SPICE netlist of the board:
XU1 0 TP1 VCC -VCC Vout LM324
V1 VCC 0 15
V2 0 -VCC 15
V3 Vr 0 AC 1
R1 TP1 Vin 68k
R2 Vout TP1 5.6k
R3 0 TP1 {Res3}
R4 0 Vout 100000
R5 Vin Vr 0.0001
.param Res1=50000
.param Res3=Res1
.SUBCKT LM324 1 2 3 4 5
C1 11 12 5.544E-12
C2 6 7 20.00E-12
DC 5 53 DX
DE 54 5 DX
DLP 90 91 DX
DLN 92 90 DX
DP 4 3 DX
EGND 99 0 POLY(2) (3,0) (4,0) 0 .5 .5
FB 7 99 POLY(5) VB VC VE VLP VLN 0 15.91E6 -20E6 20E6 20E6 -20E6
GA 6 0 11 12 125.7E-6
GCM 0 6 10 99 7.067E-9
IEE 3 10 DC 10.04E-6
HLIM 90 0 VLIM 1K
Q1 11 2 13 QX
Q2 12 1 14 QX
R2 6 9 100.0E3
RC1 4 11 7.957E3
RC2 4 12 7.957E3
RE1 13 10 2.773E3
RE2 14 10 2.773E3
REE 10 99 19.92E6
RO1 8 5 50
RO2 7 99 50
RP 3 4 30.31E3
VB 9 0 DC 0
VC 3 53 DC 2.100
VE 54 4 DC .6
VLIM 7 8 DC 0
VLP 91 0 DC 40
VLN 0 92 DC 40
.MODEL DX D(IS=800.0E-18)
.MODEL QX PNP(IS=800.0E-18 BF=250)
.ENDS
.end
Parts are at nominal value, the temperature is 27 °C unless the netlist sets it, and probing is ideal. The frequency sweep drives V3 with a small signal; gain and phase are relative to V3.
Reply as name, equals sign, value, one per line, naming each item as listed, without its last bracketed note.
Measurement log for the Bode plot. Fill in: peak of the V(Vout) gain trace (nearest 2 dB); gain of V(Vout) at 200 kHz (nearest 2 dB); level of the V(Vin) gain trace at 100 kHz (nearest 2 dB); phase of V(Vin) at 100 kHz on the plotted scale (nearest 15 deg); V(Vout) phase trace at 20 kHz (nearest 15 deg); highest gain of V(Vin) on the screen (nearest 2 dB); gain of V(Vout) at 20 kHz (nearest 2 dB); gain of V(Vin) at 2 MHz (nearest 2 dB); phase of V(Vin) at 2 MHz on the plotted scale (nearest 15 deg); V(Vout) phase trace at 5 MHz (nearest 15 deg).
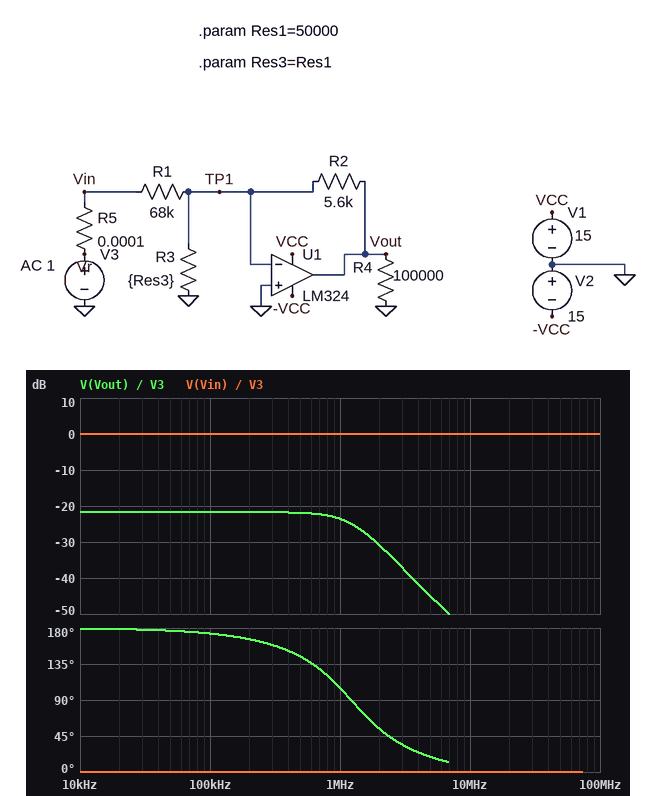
peak of the V(Vout) gain trace = -22 dB
gain of V(Vout) at 200 kHz = -22 dB
level of the V(Vin) gain trace at 100 kHz = 0 dB
phase of V(Vin) at 100 kHz on the plotted scale = 0 deg
V(Vout) phase trace at 20 kHz = 180 deg
highest gain of V(Vin) on the screen = 0 dB
gain of V(Vout) at 20 kHz = -22 dB
gain of V(Vin) at 2 MHz = 0 dB
phase of V(Vin) at 2 MHz on the plotted scale = 0 deg
V(Vout) phase trace at 5 MHz = 15 deg
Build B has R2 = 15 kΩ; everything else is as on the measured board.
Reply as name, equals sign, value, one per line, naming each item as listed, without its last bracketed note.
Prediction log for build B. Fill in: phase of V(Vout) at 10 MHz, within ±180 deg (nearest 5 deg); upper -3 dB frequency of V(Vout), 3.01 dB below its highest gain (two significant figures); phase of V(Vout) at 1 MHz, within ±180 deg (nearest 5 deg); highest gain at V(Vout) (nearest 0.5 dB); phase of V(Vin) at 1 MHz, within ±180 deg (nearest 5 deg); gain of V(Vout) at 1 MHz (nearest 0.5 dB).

phase of V(Vout) at 10 MHz, within ±180 deg = 10 deg
upper -3 dB frequency of V(Vout), 3.01 dB below its highest gain = 900 kHz
phase of V(Vout) at 1 MHz, within ±180 deg = 95 deg
highest gain at V(Vout) = -13.0 dB
phase of V(Vin) at 1 MHz, within ±180 deg = 0 deg
gain of V(Vout) at 1 MHz = -17.0 dB
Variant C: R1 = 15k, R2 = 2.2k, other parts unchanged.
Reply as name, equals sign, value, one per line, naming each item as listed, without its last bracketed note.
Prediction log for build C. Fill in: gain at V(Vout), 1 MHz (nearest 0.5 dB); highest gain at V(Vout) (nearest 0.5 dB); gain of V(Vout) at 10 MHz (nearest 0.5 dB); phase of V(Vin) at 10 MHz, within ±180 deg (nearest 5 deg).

gain at V(Vout), 1 MHz = -18.5 dB
highest gain at V(Vout) = -16.5 dB
gain of V(Vout) at 10 MHz = -46.0 dB
phase of V(Vin) at 10 MHz, within ±180 deg = 0 deg
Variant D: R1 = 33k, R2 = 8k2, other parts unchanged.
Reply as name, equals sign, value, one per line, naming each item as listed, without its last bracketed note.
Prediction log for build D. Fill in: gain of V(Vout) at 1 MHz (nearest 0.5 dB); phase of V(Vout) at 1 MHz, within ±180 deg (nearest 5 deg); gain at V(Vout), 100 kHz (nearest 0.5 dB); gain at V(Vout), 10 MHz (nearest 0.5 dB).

gain of V(Vout) at 1 MHz = -15.0 dB
phase of V(Vout) at 1 MHz, within ±180 deg = 100 deg
gain at V(Vout), 100 kHz = -12.0 dB
gain at V(Vout), 10 MHz = -47.5 dB
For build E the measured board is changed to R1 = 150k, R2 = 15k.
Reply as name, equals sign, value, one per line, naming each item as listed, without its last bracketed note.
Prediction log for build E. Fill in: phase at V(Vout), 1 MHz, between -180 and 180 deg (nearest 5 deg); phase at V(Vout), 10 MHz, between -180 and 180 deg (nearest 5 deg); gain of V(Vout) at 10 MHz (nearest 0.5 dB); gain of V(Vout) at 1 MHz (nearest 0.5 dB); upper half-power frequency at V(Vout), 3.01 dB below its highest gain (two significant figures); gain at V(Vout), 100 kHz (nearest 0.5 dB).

phase at V(Vout), 1 MHz, between -180 and 180 deg = 100 deg
phase at V(Vout), 10 MHz, between -180 and 180 deg = 10 deg
gain of V(Vout) at 10 MHz = -56.5 dB
gain of V(Vout) at 1 MHz = -23.0 dB
upper half-power frequency at V(Vout), 3.01 dB below its highest gain = 990 kHz
gain at V(Vout), 100 kHz = -20.0 dB
